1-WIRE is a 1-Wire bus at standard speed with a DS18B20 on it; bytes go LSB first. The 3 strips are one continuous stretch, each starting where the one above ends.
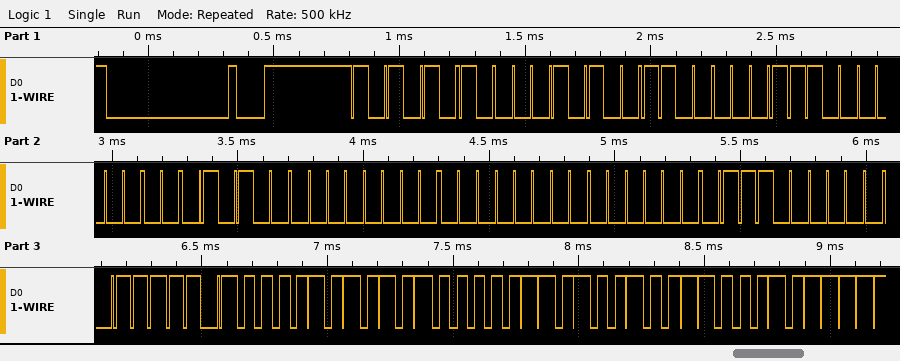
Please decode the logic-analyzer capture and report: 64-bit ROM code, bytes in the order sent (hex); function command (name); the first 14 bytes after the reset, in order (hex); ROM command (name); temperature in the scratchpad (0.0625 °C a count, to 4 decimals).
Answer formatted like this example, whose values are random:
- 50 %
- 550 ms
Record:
- 28 83 03 28 00 00 80 03
- Read Scratchpad
- 55 28 83 03 28 00 00 80 03 BE 50 05 4B 46
- Match ROM
- 85.0000 °C
